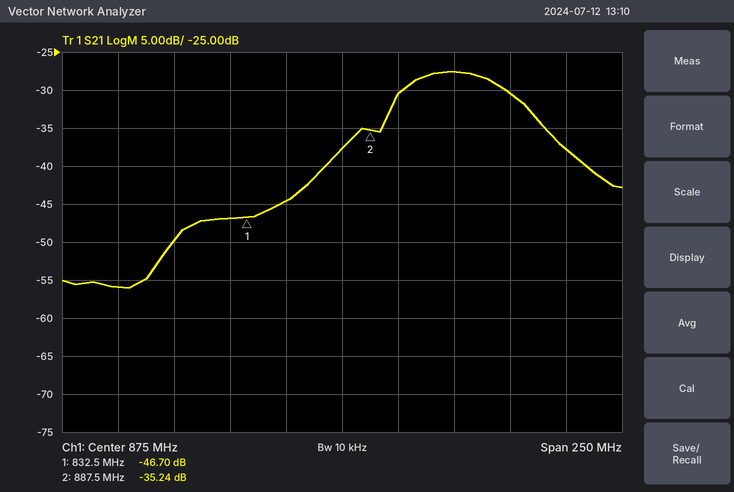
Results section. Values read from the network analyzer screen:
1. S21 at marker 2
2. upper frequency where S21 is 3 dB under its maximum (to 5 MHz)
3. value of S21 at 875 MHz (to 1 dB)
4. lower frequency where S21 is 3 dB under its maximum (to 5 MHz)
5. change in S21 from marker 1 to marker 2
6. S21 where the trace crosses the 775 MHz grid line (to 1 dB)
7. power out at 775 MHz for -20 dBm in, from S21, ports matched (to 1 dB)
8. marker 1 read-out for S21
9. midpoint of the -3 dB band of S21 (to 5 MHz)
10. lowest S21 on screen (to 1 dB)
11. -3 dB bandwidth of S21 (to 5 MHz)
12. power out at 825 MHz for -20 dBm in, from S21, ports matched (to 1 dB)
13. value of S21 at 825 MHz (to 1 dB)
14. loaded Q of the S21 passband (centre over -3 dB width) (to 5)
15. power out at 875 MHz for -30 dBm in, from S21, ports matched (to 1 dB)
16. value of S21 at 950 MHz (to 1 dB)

-35.24 dB
950 MHz
-38 dB
900 MHz
11.46 dB
-56 dB
-76 dBm
-46.70 dB
925 MHz
-56 dB
50 MHz
-67 dBm
-47 dB
20
-68 dBm
-30 dB
